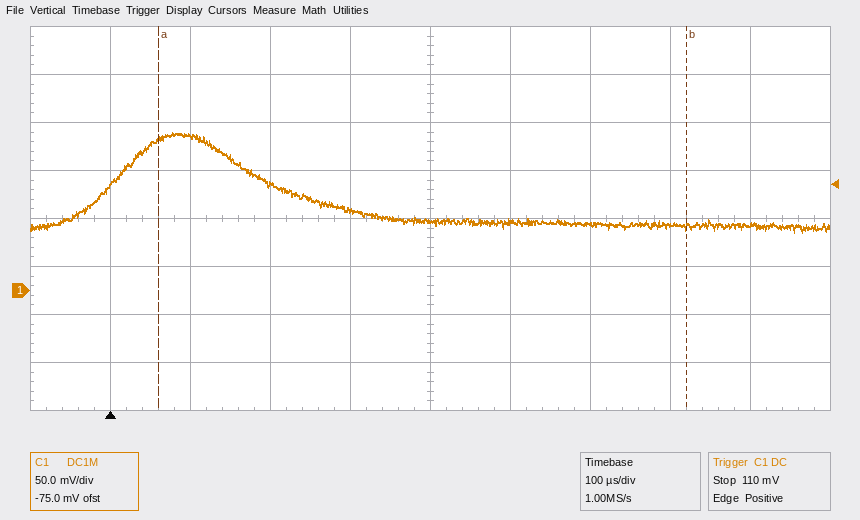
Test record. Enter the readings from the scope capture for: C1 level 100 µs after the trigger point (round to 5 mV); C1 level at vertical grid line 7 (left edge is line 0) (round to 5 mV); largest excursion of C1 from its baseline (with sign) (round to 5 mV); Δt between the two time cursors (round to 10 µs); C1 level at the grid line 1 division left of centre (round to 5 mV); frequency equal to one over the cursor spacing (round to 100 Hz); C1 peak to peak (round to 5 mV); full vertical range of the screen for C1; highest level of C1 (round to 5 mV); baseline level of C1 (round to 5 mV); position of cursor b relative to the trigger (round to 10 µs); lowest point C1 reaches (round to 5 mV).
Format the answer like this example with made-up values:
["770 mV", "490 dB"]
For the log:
["160 mV", "70 mV", "+95 mV", "660 µs", "85 mV", "1.5 kHz", "105 mV", "400 mV", "165 mV", "70 mV", "+720 µs", "60 mV"]
